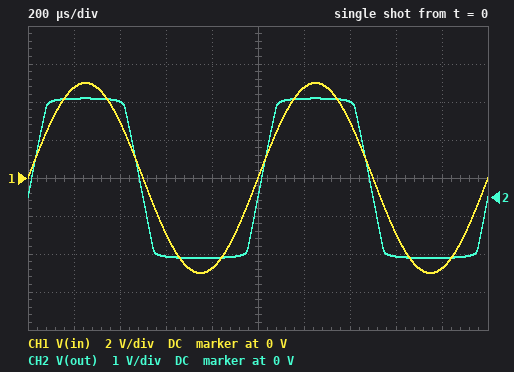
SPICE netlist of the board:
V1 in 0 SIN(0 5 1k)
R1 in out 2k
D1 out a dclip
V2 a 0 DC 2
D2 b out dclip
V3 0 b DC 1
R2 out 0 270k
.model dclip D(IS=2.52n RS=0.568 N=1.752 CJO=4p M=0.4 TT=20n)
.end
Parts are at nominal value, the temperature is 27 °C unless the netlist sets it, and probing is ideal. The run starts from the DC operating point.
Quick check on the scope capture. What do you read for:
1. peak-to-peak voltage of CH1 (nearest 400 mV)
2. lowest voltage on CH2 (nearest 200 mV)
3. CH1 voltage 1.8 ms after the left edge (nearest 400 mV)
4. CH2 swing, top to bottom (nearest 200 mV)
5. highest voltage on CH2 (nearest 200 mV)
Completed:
10.0 V
-1.6 V
-4.8 V
4.2 V
2.6 V
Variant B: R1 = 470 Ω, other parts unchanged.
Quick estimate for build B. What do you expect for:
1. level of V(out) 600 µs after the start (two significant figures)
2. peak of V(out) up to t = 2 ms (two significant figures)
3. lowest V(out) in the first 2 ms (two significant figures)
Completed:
-1.6 V
2.7 V
-1.7 V
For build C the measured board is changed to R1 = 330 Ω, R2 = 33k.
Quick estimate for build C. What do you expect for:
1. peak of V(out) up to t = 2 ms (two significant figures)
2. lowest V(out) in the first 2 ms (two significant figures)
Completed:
2.7 V
-1.7 V
